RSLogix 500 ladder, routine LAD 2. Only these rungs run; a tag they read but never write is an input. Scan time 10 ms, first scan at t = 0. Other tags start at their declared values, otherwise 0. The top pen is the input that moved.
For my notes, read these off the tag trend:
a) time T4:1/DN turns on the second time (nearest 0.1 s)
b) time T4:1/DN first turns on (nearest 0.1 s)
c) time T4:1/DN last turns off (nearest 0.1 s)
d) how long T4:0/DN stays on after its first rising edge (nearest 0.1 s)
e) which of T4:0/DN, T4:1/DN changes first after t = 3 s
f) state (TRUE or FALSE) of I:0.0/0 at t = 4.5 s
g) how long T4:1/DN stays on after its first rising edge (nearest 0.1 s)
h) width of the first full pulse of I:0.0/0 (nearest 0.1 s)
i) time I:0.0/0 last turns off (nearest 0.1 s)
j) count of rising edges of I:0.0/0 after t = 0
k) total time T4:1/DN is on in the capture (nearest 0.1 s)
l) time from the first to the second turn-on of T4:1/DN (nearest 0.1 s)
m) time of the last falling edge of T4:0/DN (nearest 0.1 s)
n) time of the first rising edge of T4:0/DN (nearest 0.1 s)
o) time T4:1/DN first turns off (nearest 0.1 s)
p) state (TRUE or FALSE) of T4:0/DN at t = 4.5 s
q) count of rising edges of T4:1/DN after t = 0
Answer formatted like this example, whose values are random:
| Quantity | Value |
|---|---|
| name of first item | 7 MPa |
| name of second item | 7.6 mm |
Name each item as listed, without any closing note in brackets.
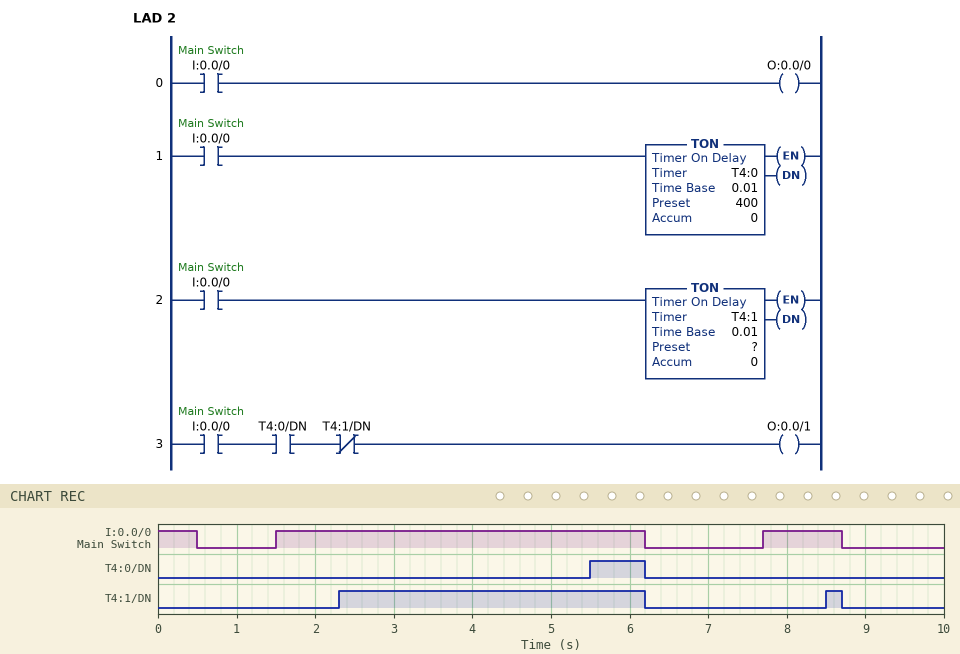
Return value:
| Quantity | Value |
|---|---|
| time T4:1/DN turns on the second time | 8.5 s |
| time T4:1/DN first turns on | 2.3 s |
| time T4:1/DN last turns off | 8.7 s |
| how long T4:0/DN stays on after its first rising edge | 0.7 s |
| which of T4:0/DN, T4:1/DN changes first after t = 3 s | T4:0/DN |
| state (TRUE or FALSE) of I:0.0/0 at t = 4.5 s | TRUE |
| how long T4:1/DN stays on after its first rising edge | 3.9 s |
| width of the first full pulse of I:0.0/0 | 4.7 s |
| time I:0.0/0 last turns off | 8.7 s |
| count of rising edges of I:0.0/0 after t = 0 | 2 |
| total time T4:1/DN is on in the capture | 4.1 s |
| time from the first to the second turn-on of T4:1/DN | 6.2 s |
| time of the last falling edge of T4:0/DN | 6.2 s |
| time of the first rising edge of T4:0/DN | 5.5 s |
| time T4:1/DN first turns off | 6.2 s |
| state (TRUE or FALSE) of T4:0/DN at t = 4.5 s | FALSE |
| count of rising edges of T4:1/DN after t = 0 | 2 |
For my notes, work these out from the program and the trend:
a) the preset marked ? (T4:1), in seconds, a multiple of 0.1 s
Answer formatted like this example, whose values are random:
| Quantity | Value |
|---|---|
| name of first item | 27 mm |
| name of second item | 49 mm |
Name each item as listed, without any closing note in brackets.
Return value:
| Quantity | Value |
|---|---|
| the preset marked ? (T4:1), in seconds, a multiple of 0.1 s | 0.8 s |
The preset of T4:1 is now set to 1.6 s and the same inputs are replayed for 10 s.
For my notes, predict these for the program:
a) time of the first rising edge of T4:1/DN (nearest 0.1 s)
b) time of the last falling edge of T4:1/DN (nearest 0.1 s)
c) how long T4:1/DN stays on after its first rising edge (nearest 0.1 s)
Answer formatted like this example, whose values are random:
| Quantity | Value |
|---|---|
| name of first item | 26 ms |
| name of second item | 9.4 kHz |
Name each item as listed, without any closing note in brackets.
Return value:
| Quantity | Value |
|---|---|
| time of the first rising edge of T4:1/DN | 3.1 s |
| time of the last falling edge of T4:1/DN | 6.2 s |
| how long T4:1/DN stays on after its first rising edge | 3.1 s |
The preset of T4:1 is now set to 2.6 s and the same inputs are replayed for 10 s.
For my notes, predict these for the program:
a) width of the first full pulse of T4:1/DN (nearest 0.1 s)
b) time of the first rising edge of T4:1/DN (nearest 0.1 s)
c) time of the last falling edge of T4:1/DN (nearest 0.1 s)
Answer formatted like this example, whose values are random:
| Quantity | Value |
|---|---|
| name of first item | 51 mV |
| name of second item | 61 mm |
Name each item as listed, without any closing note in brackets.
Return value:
| Quantity | Value |
|---|---|
| width of the first full pulse of T4:1/DN | 2.1 s |
| time of the first rising edge of T4:1/DN | 4.1 s |
| time of the last falling edge of T4:1/DN | 6.2 s |
